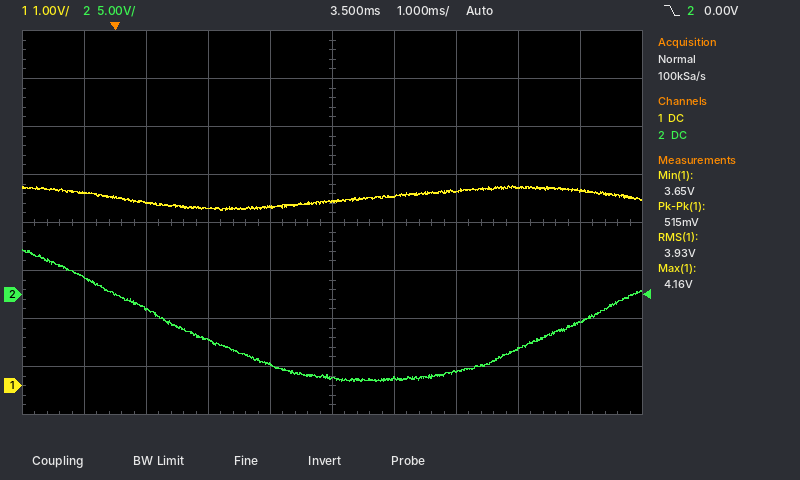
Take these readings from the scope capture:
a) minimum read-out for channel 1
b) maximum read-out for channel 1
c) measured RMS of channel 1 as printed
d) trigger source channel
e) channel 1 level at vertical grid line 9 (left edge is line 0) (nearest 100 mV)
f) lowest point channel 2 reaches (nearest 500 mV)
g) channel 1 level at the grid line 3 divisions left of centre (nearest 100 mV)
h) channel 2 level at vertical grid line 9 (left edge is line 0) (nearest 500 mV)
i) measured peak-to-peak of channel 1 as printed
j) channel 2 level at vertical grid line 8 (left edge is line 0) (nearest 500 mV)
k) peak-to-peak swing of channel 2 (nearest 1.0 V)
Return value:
3.65 V
4.16 V
3.93 V
channel 2
4.1 V
-9.0 V
3.8 V
-3.0 V
515 mV
-5.5 V
14.0 V
